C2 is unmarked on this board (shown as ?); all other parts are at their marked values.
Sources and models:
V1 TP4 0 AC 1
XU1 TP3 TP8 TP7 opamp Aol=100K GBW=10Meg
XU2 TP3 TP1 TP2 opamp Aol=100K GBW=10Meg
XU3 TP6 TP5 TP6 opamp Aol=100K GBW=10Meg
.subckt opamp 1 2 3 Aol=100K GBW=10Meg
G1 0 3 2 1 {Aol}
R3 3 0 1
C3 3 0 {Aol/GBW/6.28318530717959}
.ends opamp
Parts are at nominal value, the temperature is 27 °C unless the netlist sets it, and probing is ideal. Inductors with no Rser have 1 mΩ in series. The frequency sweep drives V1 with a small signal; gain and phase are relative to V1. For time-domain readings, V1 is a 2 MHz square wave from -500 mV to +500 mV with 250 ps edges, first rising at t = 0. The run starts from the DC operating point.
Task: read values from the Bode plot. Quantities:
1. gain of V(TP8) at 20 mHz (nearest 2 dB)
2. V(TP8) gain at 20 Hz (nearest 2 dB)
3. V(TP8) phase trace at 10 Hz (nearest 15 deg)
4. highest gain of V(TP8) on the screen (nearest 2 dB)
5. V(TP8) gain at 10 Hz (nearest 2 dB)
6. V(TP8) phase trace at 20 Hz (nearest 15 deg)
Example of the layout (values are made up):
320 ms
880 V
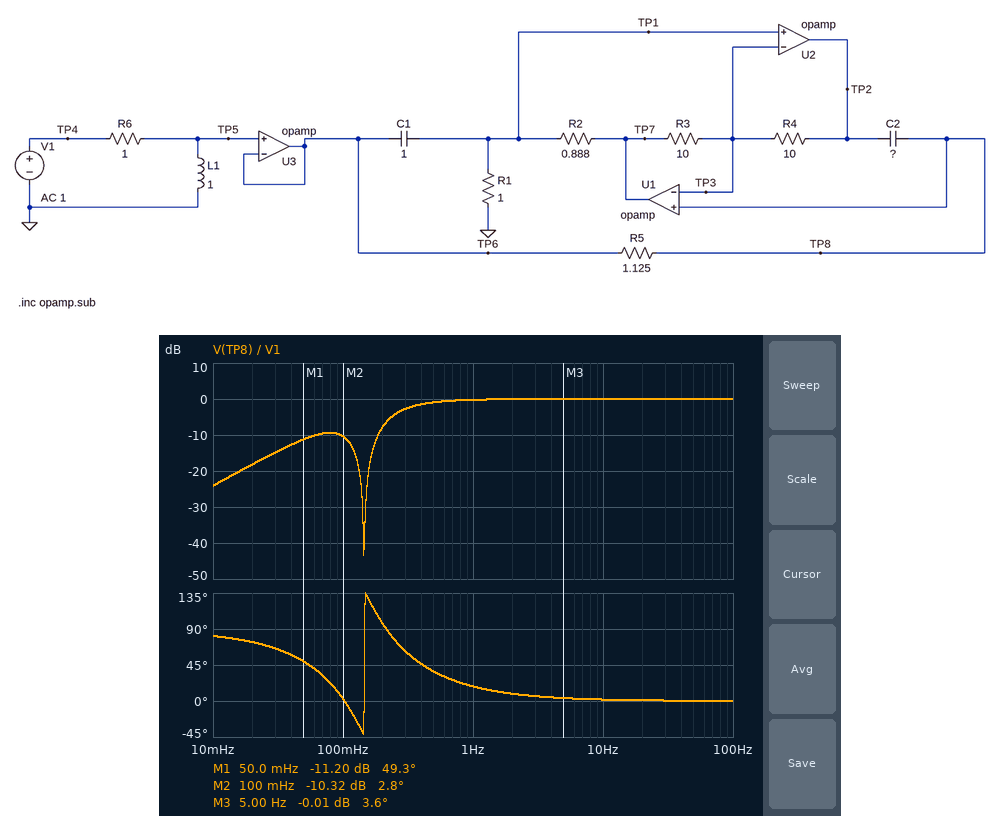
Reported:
-18 dB
0 dB
0 deg
0 dB
0 dB
0 deg
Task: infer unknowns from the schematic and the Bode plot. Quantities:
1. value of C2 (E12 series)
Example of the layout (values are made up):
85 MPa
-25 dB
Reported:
1.2 F
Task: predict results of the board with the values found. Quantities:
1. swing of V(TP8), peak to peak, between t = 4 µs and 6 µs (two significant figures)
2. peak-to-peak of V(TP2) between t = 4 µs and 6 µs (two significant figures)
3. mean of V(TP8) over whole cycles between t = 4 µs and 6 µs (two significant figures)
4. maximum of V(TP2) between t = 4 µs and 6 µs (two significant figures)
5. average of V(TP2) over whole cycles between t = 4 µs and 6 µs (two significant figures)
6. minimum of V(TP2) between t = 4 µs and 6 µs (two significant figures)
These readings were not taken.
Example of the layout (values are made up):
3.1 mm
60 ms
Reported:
1.3 V
1.3 V
500 mV
1.1 V
500 mV
-140 mV
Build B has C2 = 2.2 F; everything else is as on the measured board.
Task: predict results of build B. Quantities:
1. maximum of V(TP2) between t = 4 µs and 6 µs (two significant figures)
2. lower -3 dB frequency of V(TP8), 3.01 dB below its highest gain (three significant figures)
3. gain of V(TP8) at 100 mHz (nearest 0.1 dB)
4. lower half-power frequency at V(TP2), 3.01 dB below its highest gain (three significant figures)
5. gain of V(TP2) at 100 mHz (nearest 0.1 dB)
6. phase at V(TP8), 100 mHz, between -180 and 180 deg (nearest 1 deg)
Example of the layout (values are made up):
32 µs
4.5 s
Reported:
1.1 V
271 mHz
-25.9 dB
199 mHz
-10.8 dB
-27 deg
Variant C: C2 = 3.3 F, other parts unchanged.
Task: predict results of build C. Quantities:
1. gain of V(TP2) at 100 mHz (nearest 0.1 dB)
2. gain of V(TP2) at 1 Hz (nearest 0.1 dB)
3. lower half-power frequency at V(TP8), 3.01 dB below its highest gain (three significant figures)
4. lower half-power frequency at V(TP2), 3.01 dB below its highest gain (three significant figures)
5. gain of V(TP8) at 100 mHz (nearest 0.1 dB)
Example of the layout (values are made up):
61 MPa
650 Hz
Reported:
-10.4 dB
-0.2 dB
263 mHz
215 mHz
-22.3 dB
